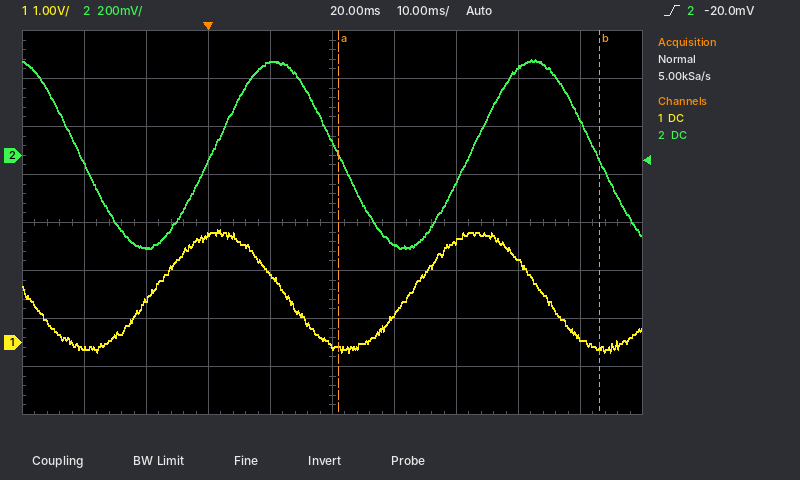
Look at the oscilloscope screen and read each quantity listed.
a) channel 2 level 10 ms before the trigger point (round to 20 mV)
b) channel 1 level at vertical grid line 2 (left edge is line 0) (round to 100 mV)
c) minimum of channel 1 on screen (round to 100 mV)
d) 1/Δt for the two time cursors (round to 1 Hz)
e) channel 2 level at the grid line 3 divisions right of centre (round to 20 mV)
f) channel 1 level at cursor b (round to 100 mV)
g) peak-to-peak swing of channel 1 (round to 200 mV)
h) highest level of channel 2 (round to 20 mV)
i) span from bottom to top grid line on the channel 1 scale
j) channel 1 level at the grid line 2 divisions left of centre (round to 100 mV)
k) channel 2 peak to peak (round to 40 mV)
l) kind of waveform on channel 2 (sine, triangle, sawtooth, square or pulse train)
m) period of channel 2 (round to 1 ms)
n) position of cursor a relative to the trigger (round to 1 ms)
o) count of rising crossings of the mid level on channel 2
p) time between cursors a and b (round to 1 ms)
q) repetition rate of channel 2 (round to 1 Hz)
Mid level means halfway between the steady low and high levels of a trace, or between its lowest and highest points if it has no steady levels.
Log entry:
-380 mV
900 mV
-200 mV
24 Hz
360 mV
-100 mV
2.6 V
400 mV
8 V
2.2 V
800 mV
sine
42 ms
+21 ms
2
42 ms
24 Hz
